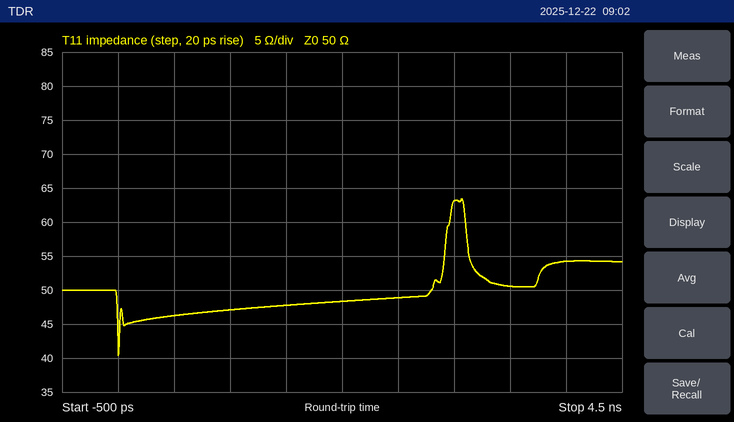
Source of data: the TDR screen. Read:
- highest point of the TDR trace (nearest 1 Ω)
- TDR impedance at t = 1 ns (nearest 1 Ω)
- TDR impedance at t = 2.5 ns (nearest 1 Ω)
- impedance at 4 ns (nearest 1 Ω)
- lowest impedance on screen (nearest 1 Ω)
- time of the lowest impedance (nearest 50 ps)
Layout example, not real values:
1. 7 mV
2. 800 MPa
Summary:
1. 63 Ω
2. 47 Ω
3. 49 Ω
4. 54 Ω
5. 40 Ω
6. 0 ps
